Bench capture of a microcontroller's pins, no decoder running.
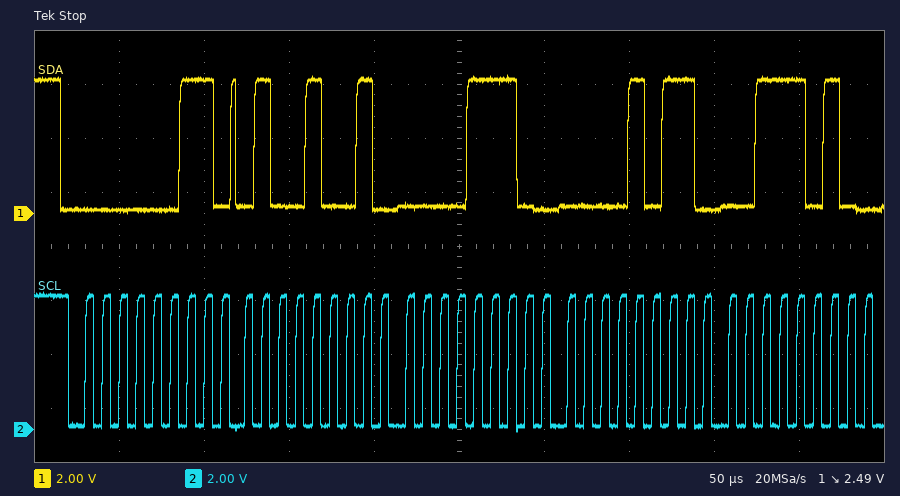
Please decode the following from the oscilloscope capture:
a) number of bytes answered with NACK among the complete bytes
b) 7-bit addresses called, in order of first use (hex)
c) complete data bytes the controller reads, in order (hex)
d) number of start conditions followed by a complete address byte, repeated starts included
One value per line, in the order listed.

0
0x01
49 0E 0B 3A
1
